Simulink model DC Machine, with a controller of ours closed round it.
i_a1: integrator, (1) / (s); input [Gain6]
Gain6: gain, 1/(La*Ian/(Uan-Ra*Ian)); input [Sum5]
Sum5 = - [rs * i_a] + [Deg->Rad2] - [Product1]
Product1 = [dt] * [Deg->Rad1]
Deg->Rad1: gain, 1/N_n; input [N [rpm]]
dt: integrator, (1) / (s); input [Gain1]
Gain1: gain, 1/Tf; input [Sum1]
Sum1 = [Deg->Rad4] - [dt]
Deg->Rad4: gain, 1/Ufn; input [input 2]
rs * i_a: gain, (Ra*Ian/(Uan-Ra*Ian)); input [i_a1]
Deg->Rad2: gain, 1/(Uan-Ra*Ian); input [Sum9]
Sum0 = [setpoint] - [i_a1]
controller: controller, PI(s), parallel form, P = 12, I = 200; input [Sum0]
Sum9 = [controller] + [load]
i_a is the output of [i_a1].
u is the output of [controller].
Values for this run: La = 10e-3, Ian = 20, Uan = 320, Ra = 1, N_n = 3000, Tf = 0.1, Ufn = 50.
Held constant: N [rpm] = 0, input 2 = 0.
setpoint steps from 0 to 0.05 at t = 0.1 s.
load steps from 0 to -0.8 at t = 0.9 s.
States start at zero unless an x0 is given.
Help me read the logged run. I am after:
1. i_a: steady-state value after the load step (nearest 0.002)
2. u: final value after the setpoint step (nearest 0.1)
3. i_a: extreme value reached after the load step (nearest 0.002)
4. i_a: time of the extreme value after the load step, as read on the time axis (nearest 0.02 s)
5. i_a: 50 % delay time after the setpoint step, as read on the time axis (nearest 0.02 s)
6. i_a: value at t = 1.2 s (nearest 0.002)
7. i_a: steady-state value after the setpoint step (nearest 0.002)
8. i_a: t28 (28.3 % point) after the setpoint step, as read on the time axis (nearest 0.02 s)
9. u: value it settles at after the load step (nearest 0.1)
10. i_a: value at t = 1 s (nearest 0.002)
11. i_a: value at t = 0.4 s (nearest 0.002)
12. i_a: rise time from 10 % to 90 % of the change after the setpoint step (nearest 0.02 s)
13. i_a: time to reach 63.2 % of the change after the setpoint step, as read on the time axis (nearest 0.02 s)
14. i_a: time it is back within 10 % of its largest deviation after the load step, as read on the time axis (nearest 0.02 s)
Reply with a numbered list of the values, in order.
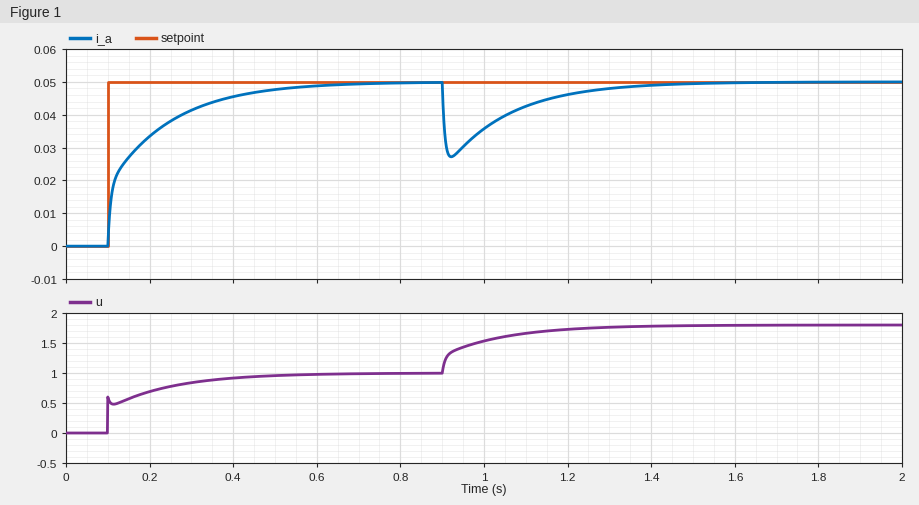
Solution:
1. 0.050
2. 1.0
3. 0.028
4. 0.92 s
5. 0.14 s
6. 0.046
7. 0.050
8. 0.10 s
9. 1.8
10. 0.036
11. 0.046
12. 0.28 s
13. 0.18 s
14. 1.28 s
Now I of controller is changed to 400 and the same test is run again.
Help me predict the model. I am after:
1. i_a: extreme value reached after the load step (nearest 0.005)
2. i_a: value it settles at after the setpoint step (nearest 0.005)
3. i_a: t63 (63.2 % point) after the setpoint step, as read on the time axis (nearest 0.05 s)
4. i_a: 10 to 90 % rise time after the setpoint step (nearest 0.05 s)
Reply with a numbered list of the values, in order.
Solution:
1. 0.030
2. 0.050
3. 0.15 s
4. 0.15 s
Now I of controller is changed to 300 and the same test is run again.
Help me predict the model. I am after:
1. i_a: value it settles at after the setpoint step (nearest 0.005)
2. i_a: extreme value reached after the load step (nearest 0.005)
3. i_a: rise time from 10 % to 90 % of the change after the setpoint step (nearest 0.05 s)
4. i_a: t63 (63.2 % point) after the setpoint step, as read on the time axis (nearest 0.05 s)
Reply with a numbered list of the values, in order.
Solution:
1. 0.050
2. 0.030
3. 0.20 s
4. 0.15 s
